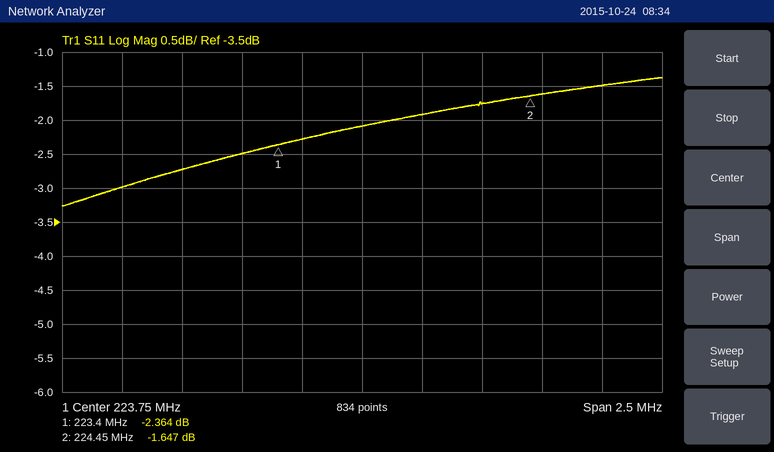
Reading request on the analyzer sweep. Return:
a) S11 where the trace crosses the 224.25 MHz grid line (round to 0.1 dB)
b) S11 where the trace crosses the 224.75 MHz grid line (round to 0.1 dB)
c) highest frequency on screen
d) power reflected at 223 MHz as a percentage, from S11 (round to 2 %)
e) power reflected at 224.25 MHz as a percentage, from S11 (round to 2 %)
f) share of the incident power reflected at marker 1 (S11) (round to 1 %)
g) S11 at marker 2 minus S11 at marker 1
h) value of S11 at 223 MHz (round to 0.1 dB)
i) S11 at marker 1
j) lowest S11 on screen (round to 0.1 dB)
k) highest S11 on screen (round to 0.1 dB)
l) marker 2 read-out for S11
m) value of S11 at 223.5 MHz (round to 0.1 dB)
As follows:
-1.8 dB
-1.5 dB
225 MHz
54 %
66 %
58 %
0.717 dB
-2.7 dB
-2.364 dB
-3.3 dB
-1.4 dB
-1.647 dB
-2.3 dB
